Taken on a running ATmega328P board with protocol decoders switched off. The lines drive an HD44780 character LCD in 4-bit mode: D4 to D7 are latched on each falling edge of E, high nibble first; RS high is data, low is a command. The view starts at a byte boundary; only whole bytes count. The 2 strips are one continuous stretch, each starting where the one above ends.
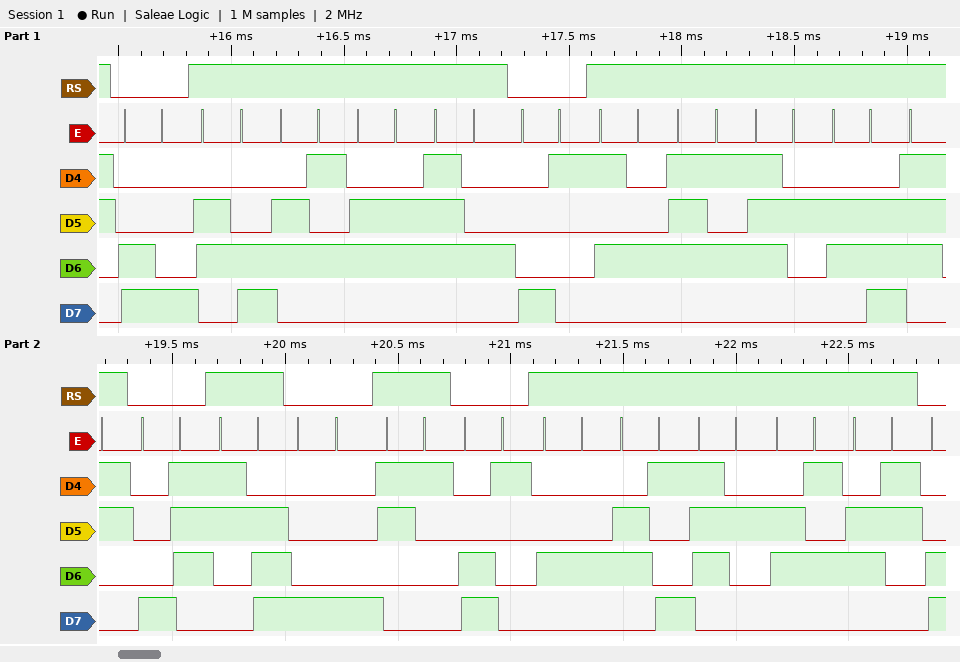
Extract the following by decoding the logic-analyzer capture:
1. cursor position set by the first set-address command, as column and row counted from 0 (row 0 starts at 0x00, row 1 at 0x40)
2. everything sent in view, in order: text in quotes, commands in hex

column 8, row 1
0xC8 "left" 0x81 "Turns" 0x87 ">" 0x88 "1" 0xC1 "Direc"
